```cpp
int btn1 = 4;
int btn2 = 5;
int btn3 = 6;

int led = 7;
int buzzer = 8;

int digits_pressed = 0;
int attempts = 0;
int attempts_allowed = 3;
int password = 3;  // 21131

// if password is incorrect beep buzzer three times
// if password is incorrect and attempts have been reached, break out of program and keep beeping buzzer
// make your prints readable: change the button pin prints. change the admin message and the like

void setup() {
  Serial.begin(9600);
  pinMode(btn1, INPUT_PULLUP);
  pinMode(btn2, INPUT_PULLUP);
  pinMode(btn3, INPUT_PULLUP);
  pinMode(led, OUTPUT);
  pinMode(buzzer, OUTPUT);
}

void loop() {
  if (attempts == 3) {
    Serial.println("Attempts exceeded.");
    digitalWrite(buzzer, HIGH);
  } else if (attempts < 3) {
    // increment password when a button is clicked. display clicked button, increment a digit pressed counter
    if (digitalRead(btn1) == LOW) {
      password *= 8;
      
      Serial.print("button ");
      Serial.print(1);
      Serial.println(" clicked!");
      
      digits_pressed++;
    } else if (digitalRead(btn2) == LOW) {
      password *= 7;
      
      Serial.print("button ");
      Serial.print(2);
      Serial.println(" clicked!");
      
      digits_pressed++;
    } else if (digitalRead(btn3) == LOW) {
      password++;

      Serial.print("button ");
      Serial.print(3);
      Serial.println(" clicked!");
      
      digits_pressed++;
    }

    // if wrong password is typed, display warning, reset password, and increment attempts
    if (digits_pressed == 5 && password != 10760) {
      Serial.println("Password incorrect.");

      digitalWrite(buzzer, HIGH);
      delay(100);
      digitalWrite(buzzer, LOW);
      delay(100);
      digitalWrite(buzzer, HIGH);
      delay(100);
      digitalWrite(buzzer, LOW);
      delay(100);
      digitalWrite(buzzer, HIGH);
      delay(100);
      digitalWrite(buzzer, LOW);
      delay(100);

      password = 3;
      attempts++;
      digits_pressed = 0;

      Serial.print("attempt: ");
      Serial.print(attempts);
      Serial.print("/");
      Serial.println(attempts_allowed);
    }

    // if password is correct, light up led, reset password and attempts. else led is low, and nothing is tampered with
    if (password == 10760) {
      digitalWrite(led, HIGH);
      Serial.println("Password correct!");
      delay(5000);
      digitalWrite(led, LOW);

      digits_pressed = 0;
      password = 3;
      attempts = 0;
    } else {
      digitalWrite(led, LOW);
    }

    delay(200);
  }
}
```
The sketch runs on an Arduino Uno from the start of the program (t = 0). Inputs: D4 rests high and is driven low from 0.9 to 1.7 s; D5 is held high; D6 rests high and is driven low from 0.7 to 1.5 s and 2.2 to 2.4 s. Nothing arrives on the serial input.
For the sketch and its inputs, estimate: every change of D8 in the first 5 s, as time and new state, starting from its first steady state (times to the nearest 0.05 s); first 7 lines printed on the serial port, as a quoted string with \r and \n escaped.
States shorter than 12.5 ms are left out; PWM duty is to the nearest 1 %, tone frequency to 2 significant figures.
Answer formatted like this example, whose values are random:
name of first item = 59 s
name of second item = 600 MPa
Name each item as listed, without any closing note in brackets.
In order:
every change of D8 in the first 5 s, as time and new state, starting from its first steady state = 0 s low; 1.6 s high; 1.7 s low; 1.8 s high; 1.9 s low; 2 s high; 2.1 s low
first 7 lines printed on the serial port, as a quoted string with \r and \n escaped = "button 3 clicked!\r\nbutton 1 clicked!\r\nbutton 1 clicked!\r\nbutton 1 clicked!\r\nbutton 1 clicked!\r\nPassword incorrect.\r\nattempt: 1/3\r\n"
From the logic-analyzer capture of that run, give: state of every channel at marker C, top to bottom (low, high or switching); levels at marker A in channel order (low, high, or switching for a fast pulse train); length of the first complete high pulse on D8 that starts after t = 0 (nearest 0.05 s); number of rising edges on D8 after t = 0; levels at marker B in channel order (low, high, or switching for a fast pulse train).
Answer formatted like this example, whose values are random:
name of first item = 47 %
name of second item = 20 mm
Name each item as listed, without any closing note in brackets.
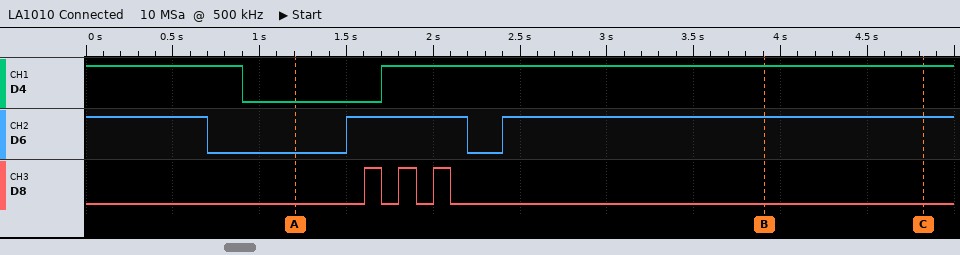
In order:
state of every channel at marker C, top to bottom = D4 high, D6 high, D8 low
levels at marker A in channel order = D4 low, D6 low, D8 low
length of the first complete high pulse on D8 that starts after t = 0 = 0.10 s
number of rising edges on D8 after t = 0 = 3
levels at marker B in channel order = D4 high, D6 high, D8 low
